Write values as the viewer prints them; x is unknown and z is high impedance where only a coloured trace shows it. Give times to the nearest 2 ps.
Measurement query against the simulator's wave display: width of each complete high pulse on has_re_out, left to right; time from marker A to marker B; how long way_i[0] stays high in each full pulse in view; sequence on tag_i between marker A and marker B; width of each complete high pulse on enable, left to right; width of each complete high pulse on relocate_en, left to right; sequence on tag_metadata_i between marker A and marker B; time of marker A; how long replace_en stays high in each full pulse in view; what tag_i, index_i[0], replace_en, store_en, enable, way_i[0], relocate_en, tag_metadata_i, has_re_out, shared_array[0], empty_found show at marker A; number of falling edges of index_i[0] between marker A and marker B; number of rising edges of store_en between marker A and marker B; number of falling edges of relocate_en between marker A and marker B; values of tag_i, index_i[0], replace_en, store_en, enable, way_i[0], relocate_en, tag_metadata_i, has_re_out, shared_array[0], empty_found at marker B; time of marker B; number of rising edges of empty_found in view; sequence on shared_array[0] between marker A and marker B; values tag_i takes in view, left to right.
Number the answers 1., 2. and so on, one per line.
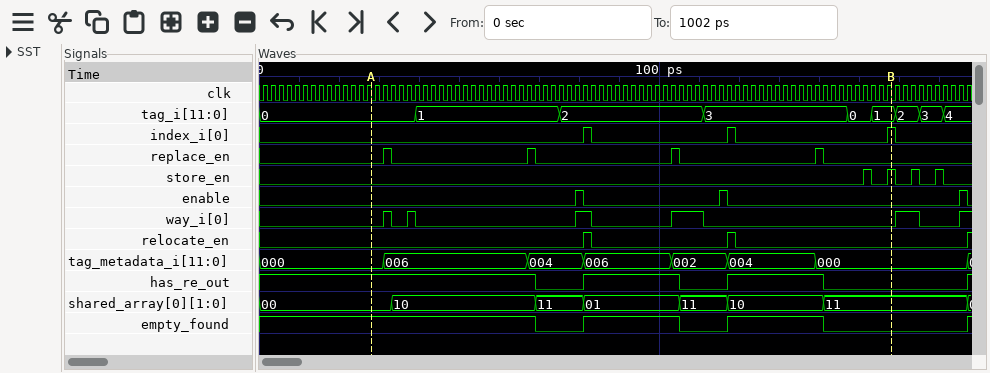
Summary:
1. 24 ps, 24 ps
2. 130 ps
3. 2 ps, 2 ps, 4 ps, 8 ps, 6 ps
4. 0, 1, 2, 3, 0, 1
5. 2 ps, 2 ps, 2 ps
6. 2 ps, 2 ps
7. 000, 006, 004, 006, 002, 004, 000
8. 28 ps
9. 2 ps, 2 ps, 2 ps, 2 ps
10. tag_i=0, index_i[0]=0, replace_en=0, store_en=0, enable=0, way_i[0]=0, relocate_en=0, tag_metadata_i=000, has_re_out=1, shared_array[0]=00, empty_found=1
11. 2
12. 2
13. 2
14. tag_i=1, index_i[0]=1, replace_en=0, store_en=1, enable=0, way_i[0]=0, relocate_en=0, tag_metadata_i=000, has_re_out=0, shared_array[0]=11, empty_found=0
15. 158 ps
16. 3
17. 00, 10, 11, 01, 11, 10, 11
18. 0, 1, 2, 3, 0, 1, 2, 3, 4
